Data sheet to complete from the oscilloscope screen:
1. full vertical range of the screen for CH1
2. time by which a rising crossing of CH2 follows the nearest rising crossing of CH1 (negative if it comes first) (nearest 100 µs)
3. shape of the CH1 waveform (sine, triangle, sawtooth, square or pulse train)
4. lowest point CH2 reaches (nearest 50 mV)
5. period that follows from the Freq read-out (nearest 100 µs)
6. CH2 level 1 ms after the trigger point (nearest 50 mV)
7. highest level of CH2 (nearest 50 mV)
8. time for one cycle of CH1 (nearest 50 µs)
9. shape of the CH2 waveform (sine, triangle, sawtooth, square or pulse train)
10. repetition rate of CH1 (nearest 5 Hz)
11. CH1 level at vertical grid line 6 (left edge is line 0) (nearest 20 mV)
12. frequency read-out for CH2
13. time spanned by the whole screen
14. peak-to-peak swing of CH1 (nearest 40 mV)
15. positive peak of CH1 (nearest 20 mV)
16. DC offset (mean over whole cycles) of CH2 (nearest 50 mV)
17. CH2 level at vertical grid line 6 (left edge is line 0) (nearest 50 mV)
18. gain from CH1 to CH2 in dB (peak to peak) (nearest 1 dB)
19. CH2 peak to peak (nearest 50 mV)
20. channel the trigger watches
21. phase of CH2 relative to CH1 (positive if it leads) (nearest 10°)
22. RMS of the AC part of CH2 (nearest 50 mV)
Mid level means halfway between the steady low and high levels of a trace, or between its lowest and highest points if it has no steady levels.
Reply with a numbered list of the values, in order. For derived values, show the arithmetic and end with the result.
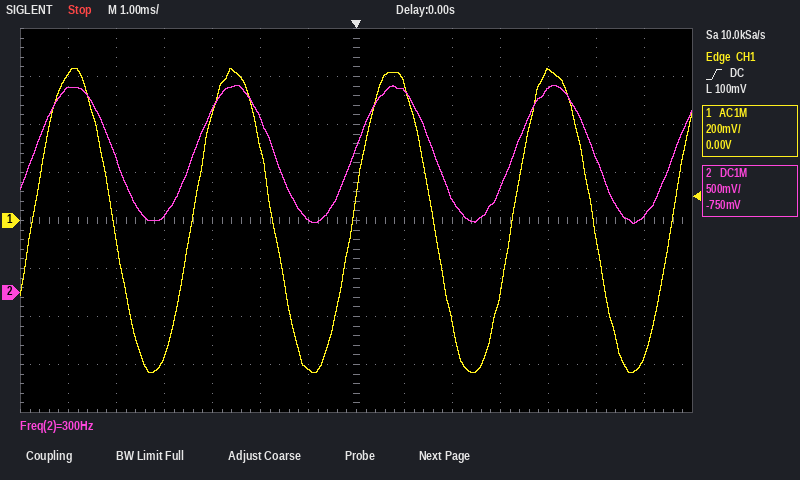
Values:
1. 1.6 V
2. 0.0 ms
3. sine
4. 700 mV
5. 1 / 300 Hz ≈ 3.3 ms
6. 2.10 V
7. 2.15 V
8. 3.35 ms
9. sine
10. 1 / 3.35 ms ≈ 299 Hz, so 300 Hz to the nearest 5 Hz
11. -620 mV
12. 300 Hz
13. 14 ms
14. 1.28 V
15. 640 mV
16. (2.15 V + (700 mV)) / 2 ≈ 1.43 V, so 1.45 V to the nearest 50 mV
17. 750 mV
18. 20 log10(1.45 V / 1.28 V) ≈ 1 dB
19. 2.15 V − (700 mV) = 1.45 V
20. CH1
21. −360° × (0.0 ms) / 3.35 ms ≈ 0°
22. 1.45 V / (2√2) ≈ 513 mV, so 500 mV to the nearest 50 mV
